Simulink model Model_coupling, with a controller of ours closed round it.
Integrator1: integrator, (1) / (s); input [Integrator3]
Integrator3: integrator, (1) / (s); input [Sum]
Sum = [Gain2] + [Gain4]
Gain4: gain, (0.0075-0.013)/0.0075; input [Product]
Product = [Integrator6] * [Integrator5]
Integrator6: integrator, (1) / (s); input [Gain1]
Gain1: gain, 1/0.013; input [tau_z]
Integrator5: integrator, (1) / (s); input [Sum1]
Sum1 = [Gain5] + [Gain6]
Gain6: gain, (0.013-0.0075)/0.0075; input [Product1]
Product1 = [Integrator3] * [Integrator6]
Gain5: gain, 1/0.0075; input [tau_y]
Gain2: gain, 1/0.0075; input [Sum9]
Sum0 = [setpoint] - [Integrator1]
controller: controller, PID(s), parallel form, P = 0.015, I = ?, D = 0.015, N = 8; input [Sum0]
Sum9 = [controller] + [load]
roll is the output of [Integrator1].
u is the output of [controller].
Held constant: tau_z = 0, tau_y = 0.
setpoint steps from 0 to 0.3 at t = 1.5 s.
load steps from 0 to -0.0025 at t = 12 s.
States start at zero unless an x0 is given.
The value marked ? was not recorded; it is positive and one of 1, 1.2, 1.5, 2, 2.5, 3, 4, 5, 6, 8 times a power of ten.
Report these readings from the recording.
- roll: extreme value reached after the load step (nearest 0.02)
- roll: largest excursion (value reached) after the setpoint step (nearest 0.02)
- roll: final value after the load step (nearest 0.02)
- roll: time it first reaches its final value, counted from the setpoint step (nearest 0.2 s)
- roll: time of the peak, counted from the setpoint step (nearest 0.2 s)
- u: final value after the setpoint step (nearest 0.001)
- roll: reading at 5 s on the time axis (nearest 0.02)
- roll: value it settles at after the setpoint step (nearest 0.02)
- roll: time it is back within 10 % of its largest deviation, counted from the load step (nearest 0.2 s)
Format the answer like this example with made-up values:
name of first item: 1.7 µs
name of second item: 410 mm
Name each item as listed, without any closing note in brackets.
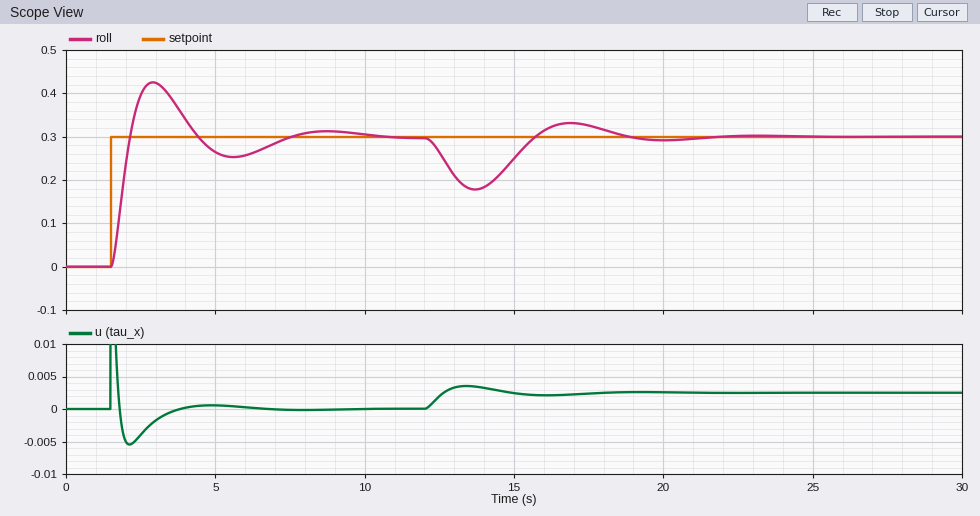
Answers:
roll: extreme value reached after the load step: 0.18
roll: largest excursion (value reached) after the setpoint step: 0.42
roll: final value after the load step: 0.30
roll: time it first reaches its final value, counted from the setpoint step: 0.6 s
roll: time of the peak, counted from the setpoint step: 1.4 s
u: final value after the setpoint step: 0.000
roll: reading at 5 s on the time axis: 0.26
roll: value it settles at after the setpoint step: 0.30
roll: time it is back within 10 % of its largest deviation, counted from the load step: 6.2 s
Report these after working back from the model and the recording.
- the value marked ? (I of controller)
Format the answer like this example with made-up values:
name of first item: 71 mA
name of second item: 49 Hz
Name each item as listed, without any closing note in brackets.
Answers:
the value marked ?: 0.012
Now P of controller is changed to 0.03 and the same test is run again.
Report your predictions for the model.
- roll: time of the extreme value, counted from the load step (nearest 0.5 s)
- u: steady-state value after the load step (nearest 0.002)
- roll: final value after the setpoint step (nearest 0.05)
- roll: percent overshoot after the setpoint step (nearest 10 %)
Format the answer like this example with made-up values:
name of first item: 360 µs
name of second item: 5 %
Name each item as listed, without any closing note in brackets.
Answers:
roll: time of the extreme value, counted from the load step: 1.5 s
u: steady-state value after the load step: 0.002
roll: final value after the setpoint step: 0.30
roll: percent overshoot after the setpoint step: 50 %
